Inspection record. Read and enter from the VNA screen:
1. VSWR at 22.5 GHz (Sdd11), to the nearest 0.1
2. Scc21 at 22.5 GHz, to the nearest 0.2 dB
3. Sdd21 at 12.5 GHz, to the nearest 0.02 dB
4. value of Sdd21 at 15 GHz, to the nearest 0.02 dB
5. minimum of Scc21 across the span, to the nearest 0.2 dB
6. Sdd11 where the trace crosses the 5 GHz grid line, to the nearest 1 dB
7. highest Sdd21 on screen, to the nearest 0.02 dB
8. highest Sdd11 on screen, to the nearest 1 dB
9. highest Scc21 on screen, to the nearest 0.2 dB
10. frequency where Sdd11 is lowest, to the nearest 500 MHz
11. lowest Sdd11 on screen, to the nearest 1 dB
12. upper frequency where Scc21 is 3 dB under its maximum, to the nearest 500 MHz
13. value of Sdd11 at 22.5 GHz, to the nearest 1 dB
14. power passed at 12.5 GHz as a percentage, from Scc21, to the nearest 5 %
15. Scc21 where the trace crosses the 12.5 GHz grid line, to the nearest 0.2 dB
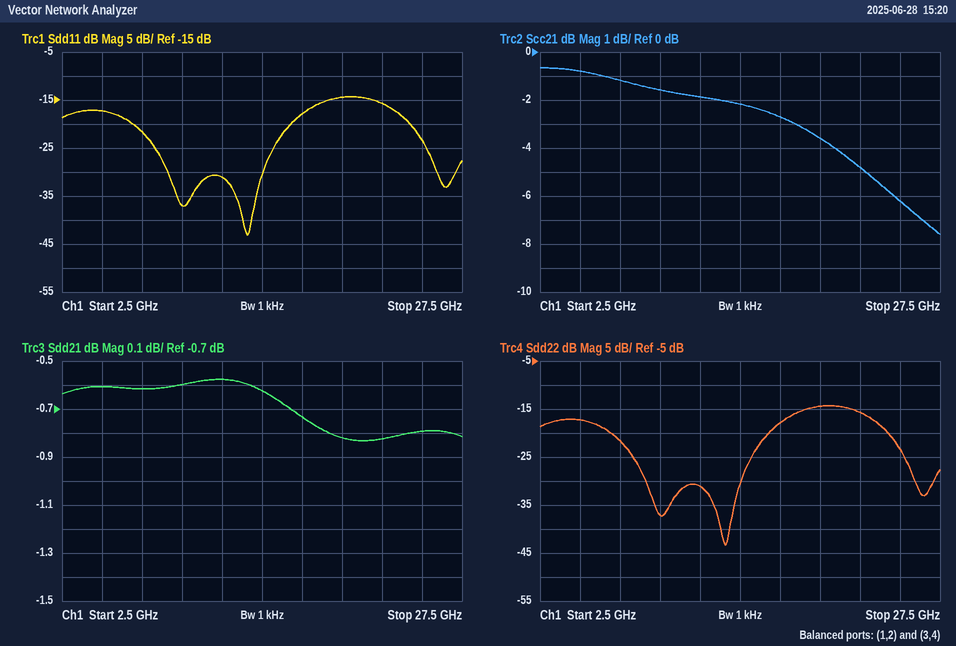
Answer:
1.4
-4.8 dB
-0.58 dB
-0.62 dB
-7.6 dB
-17 dB
-0.58 dB
-14 dB
-0.6 dB
14.0 GHz
-43 dB
20.0 GHz
-16 dB
65 %
-1.8 dB
